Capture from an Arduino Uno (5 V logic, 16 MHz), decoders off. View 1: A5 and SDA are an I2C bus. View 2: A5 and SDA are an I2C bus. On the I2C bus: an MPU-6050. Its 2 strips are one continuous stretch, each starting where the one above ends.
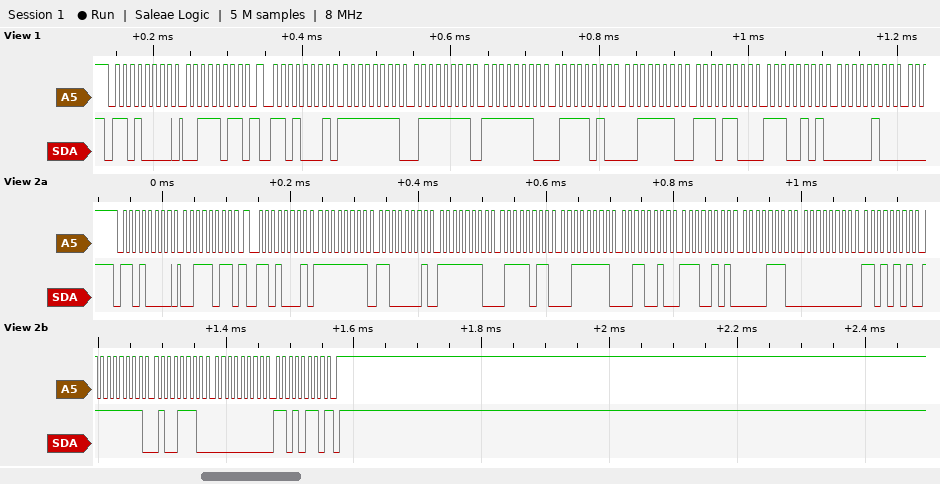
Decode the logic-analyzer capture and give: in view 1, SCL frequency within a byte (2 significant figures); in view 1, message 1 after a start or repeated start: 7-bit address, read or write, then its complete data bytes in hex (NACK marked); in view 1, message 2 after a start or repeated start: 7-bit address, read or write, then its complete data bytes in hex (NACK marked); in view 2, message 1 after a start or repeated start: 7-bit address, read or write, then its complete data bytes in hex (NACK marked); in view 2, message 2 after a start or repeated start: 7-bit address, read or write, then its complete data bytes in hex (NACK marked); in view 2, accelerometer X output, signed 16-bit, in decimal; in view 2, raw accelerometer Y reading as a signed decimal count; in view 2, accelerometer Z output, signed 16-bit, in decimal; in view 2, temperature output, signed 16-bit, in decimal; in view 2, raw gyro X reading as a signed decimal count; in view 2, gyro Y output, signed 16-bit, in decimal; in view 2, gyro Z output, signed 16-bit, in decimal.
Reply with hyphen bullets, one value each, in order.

- 100 kHz
- 0x68 write: 3B
- 0x68 read: FF 7F FE 7A 3E EC E5 04
- 0x68 write: 3B
- 0x68 read: FF C1 FE 7B 3F 32 E5 0E 00 D5 FF 4E 00 D6 NACK
- -63
- -389
- 16178
- -6898
- 213
- -178
- 214
